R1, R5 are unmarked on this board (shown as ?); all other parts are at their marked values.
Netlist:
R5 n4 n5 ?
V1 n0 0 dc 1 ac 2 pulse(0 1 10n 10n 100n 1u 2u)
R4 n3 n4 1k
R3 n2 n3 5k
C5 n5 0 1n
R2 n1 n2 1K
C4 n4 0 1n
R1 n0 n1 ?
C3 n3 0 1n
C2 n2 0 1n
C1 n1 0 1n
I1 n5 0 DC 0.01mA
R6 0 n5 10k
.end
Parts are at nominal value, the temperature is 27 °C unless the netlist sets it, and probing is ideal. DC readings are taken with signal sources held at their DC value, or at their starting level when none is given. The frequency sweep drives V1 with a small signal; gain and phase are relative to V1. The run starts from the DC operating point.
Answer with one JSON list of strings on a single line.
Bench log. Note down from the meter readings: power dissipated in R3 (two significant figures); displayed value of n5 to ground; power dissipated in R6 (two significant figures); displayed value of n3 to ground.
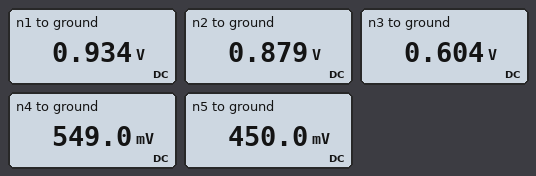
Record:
["15 µW", "450.0 mV", "20 µW", "0.604 V"]
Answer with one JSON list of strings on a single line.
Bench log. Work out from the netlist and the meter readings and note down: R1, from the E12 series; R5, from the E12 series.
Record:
["1.2 kΩ", "1.8 kΩ"]
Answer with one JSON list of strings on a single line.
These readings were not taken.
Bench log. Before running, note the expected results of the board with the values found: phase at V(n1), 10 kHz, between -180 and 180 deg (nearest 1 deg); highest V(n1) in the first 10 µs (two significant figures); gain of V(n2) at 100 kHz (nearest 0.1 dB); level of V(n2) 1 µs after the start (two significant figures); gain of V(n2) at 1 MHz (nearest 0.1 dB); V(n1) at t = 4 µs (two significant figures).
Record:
["-10 deg", "600 mV", "-8.0 dB", "160 mV", "-34.2 dB", "240 mV"]
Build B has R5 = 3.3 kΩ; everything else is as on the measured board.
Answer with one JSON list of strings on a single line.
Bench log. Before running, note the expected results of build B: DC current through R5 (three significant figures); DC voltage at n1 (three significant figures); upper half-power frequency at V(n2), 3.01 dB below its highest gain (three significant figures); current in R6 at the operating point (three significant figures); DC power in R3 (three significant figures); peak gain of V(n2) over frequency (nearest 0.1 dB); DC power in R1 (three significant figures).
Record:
["51.2 µA", "939 mV", "36.3 kHz", "41.2 µA", "13.1 µW", "-0.9 dB", "3.14 µW"]
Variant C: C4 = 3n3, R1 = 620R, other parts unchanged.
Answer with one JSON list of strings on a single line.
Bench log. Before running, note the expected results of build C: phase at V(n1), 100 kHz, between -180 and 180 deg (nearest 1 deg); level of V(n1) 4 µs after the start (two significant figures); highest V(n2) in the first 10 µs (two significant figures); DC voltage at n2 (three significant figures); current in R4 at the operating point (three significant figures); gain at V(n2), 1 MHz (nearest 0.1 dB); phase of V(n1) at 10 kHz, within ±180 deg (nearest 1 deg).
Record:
["-27 deg", "190 mV", "490 mV", "908 mV", "56.6 µA", "-28.8 dB", "-5 deg"]
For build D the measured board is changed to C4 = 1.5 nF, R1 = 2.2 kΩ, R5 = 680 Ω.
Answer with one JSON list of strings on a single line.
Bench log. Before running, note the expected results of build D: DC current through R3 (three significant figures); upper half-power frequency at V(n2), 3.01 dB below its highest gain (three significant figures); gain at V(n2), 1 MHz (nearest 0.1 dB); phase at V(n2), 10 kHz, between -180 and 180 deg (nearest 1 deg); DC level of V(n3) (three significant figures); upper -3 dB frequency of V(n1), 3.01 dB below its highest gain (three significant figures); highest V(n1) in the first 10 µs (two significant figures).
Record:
["55.3 µA", "20.7 kHz", "-39.4 dB", "-22 deg", "546 mV", "30.3 kHz", "470 mV"]
